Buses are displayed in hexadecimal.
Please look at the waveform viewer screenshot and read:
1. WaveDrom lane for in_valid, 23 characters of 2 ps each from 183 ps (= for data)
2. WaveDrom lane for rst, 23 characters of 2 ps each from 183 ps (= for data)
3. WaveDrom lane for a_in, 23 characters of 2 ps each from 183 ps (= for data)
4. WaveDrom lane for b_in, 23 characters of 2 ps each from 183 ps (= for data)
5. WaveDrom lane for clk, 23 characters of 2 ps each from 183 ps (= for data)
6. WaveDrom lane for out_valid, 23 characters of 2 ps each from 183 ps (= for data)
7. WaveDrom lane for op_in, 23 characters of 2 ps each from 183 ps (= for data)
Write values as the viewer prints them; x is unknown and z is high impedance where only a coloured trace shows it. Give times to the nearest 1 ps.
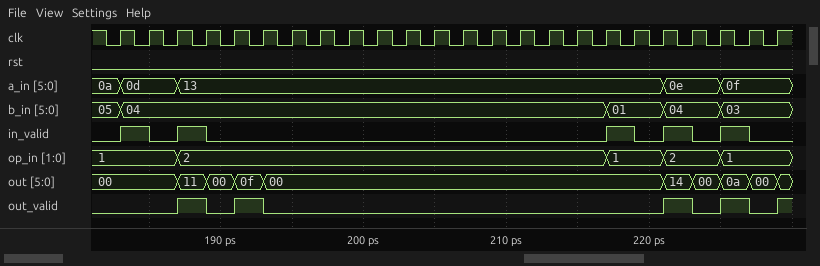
{name: 'in_valid', wave: '1010.............101010'}
{name: 'rst', wave: '0......................'}
{name: 'a_in', wave: '=.=................=.=.', data: '0d 13 0e 0f'}
{name: 'b_in', wave: '=................=.=.=.', data: '04 01 04 03'}
{name: 'clk', wave: 'p......................'}
{name: 'out_valid', wave: '0.1010.............1010'}
{name: 'op_in', wave: '=.=..............=.=.=.', data: '1 2 1 2 1'}
